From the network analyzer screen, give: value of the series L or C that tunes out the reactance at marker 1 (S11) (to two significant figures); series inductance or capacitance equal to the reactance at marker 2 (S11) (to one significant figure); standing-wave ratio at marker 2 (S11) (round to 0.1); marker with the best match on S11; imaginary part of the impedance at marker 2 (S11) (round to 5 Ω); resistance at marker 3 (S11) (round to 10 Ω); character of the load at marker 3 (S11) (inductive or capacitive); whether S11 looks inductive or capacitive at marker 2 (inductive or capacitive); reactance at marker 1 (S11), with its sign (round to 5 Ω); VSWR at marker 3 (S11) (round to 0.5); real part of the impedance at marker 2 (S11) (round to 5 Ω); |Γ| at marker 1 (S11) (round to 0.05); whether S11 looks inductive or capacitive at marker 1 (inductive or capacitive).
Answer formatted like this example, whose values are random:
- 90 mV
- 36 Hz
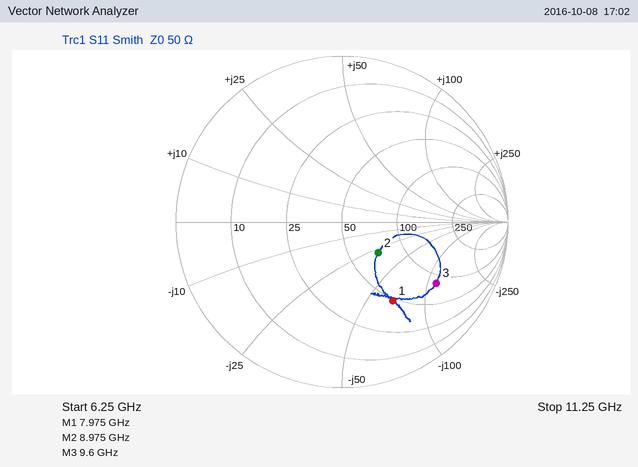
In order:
- 1.3 nH
- 600 fF
- 1.8
- marker 2
- -30 Ω
- 80 Ω
- capacitive
- capacitive
- -65 Ω
- 5.0
- 70 Ω
- 0.55
- capacitive
